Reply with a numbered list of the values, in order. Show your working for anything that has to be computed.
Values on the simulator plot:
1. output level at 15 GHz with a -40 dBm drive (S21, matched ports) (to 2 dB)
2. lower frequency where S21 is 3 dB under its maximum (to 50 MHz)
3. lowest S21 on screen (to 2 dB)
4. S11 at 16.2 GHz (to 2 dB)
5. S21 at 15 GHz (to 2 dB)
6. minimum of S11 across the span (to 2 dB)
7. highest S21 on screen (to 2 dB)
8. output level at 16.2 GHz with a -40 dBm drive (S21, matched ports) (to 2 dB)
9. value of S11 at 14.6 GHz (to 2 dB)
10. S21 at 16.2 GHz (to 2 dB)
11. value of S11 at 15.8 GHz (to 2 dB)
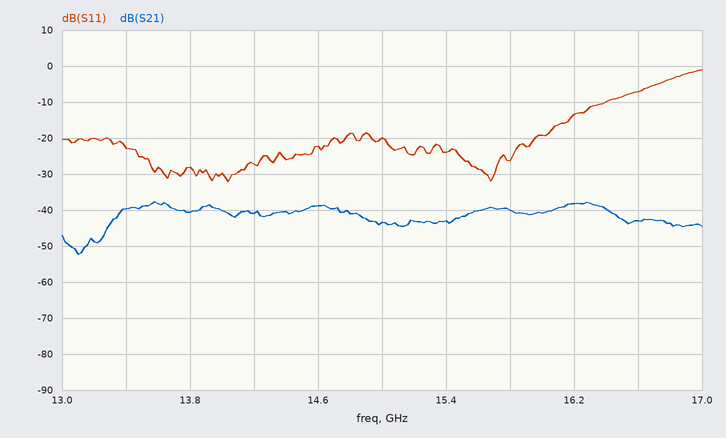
1. -40 dBm + (-44 dB) = -84 dBm
2. 13.35 GHz
3. -52 dB
4. -14 dB
5. -44 dB
6. -32 dB
7. -38 dB
8. -40 dBm + (-38 dB) = -78 dBm
9. -22 dB
10. -38 dB
11. -26 dB
